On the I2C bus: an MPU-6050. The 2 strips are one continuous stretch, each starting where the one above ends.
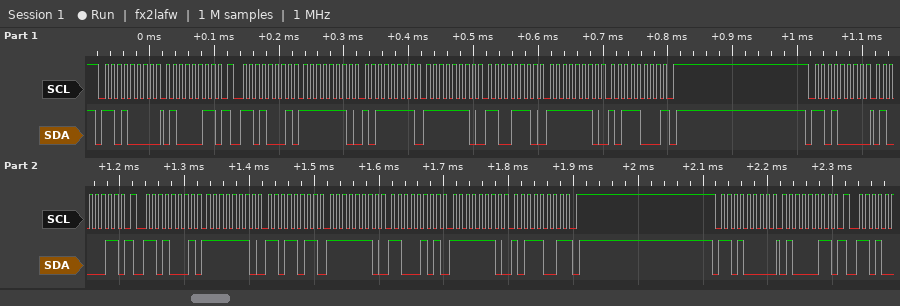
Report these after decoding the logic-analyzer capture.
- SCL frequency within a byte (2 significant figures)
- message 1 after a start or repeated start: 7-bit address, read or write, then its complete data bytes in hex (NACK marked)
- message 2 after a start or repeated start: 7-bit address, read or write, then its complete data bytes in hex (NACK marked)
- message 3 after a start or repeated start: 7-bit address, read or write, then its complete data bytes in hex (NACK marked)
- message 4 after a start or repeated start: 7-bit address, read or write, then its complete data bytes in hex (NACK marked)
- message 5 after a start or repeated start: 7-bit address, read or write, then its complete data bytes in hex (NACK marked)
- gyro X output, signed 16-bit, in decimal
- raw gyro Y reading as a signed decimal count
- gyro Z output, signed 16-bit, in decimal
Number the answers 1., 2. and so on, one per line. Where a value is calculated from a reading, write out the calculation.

1. 100 kHz
2. 0x68 write: 43
3. 0x68 read: FE BF FE CE FE B8 NACK
4. 0x68 write: 43
5. 0x68 read: FE DB FE C5 FE B9 NACK
6. 0x68 write: 43
7. 0xFEBF = -321
8. 0xFECE = -306
9. 0xFEB8 = -328
